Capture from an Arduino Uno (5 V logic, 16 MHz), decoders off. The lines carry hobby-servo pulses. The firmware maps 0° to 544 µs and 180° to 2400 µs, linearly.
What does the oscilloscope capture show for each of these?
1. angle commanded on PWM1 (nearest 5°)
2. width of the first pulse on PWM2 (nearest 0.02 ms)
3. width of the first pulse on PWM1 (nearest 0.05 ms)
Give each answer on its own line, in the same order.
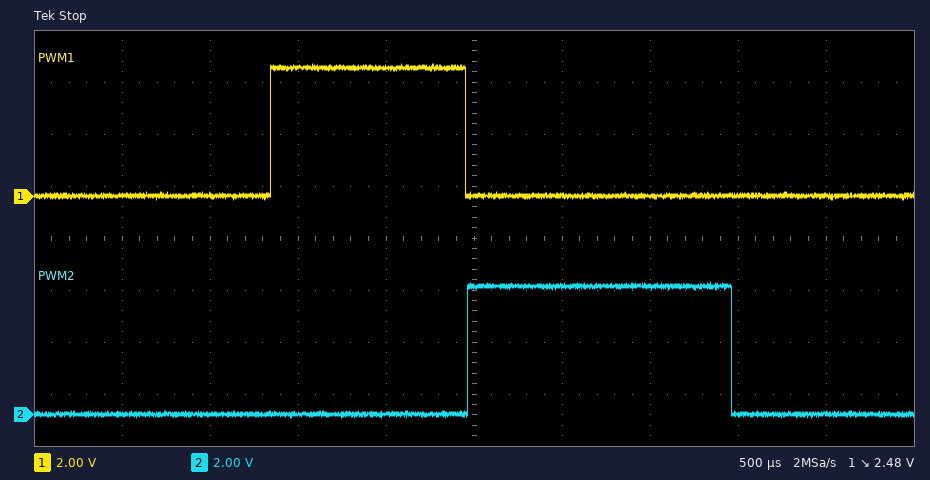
55°
1.50 ms
1.10 ms
